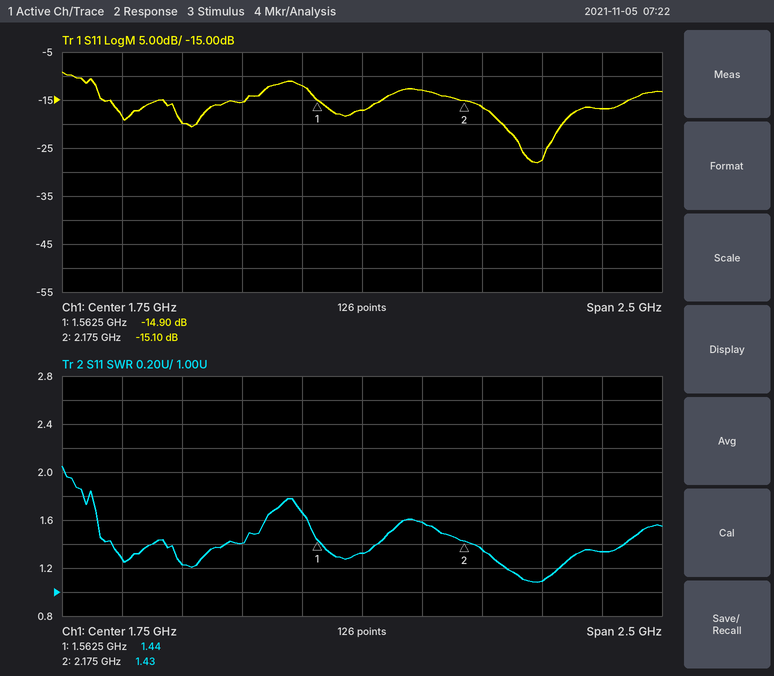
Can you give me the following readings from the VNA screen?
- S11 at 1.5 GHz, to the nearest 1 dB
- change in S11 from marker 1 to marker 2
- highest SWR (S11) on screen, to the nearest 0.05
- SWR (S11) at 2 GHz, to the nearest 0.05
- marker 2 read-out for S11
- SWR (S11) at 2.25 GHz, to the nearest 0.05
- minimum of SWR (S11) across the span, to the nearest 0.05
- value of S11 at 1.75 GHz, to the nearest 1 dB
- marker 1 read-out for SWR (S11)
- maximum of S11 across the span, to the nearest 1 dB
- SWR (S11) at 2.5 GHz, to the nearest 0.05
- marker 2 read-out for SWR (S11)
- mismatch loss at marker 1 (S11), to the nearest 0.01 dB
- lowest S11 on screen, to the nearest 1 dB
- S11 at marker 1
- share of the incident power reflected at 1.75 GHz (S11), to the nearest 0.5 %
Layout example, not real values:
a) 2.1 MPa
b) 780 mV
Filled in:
a) -12 dB
b) -0.20 dB
c) 2.05
d) 1.60
e) -15.10 dB
f) 1.35
g) 1.10
h) -17 dB
i) 1.44
j) -9 dB
k) 1.10
l) 1.43
m) 0.14 dB
n) -28 dB
o) -14.90 dB
p) 2.0 %
